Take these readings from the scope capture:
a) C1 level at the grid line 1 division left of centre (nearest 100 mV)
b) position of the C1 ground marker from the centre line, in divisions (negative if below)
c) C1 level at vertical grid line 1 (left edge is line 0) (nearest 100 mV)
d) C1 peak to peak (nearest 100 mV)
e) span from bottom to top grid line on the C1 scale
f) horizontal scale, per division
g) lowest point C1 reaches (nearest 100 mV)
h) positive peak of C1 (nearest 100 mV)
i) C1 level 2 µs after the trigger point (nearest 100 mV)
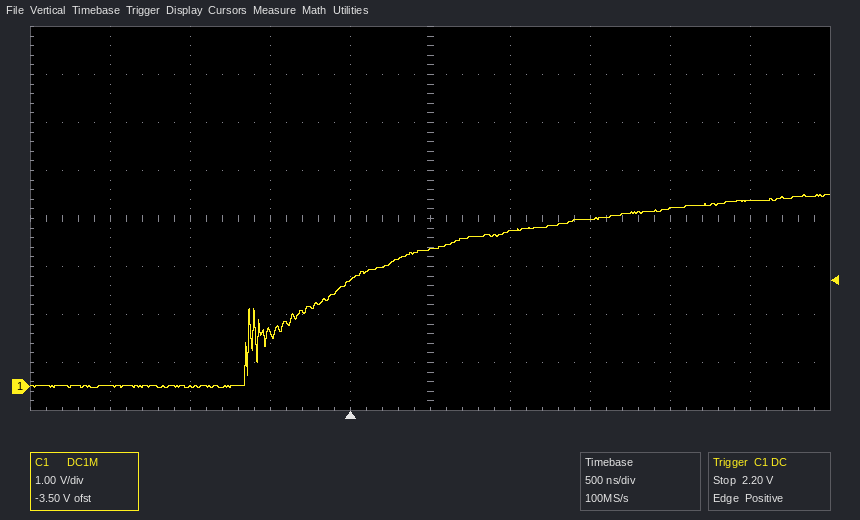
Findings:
2.2 V
-3.5 div
0.0 V
4.0 V
8 V
500 ns
0.0 V
4.0 V
3.7 V
